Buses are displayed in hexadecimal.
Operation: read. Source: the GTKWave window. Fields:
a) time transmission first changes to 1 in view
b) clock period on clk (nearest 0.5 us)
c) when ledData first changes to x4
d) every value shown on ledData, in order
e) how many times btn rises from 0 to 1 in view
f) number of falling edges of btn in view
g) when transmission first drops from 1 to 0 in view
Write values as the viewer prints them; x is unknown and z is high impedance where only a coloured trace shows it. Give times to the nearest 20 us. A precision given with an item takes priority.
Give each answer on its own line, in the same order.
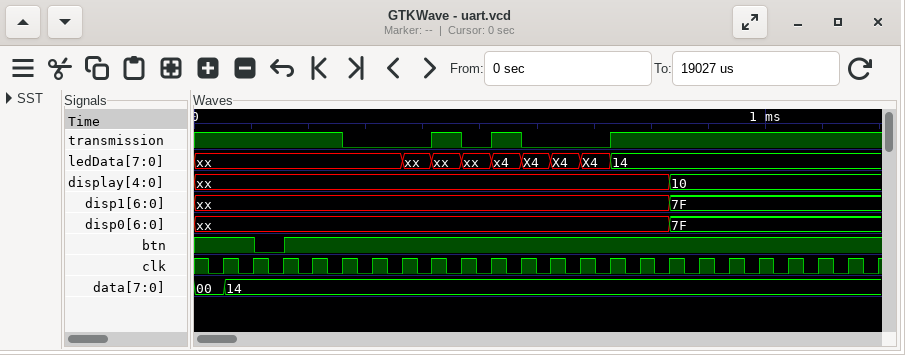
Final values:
420 us
52 us
520 us
xx, xx, xx, xx, x4, X4, X4, X4, 14
1
1
260 us
